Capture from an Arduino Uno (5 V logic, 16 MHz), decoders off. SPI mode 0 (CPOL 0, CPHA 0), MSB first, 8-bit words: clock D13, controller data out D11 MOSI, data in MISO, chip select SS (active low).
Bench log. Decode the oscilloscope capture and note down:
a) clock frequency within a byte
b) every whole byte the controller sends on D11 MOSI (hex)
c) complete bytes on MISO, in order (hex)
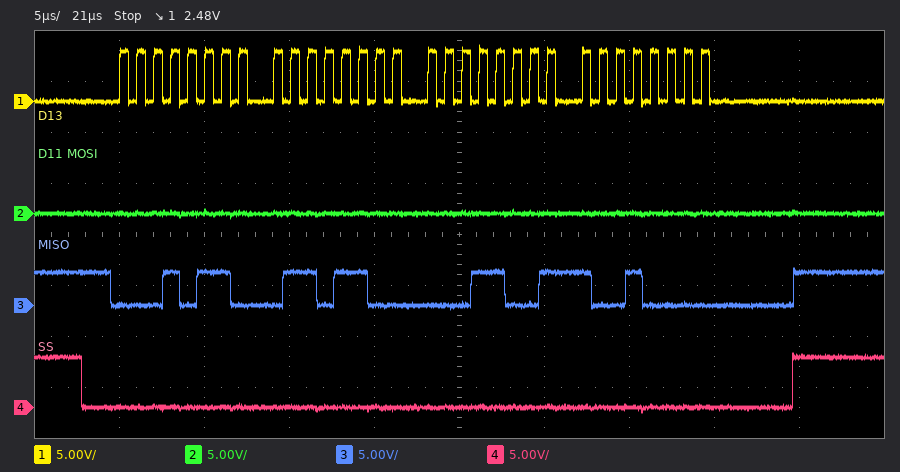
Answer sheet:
1 MHz
00 00 00 00
16 6C 19 90
